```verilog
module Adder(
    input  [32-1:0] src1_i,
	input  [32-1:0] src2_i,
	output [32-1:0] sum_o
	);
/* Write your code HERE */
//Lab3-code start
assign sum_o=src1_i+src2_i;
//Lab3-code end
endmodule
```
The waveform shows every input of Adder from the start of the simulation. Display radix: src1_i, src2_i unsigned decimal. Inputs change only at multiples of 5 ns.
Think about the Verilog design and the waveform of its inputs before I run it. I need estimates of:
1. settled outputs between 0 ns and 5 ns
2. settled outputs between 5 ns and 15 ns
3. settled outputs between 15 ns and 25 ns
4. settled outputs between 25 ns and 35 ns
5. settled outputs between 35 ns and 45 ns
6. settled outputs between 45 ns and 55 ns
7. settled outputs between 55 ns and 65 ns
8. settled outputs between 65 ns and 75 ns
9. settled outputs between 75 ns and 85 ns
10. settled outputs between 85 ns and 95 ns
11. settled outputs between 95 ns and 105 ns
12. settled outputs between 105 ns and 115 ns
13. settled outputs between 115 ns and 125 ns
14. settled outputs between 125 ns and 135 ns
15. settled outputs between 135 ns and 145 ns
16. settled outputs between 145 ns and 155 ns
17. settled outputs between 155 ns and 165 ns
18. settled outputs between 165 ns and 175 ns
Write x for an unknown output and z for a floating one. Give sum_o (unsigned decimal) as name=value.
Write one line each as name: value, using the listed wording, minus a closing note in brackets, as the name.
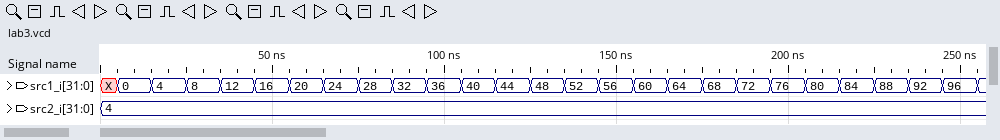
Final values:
settled outputs between 0 ns and 5 ns: sum_o=x
settled outputs between 5 ns and 15 ns: sum_o=4
settled outputs between 15 ns and 25 ns: sum_o=8
settled outputs between 25 ns and 35 ns: sum_o=12
settled outputs between 35 ns and 45 ns: sum_o=16
settled outputs between 45 ns and 55 ns: sum_o=20
settled outputs between 55 ns and 65 ns: sum_o=24
settled outputs between 65 ns and 75 ns: sum_o=28
settled outputs between 75 ns and 85 ns: sum_o=32
settled outputs between 85 ns and 95 ns: sum_o=36
settled outputs between 95 ns and 105 ns: sum_o=40
settled outputs between 105 ns and 115 ns: sum_o=44
settled outputs between 115 ns and 125 ns: sum_o=48
settled outputs between 125 ns and 135 ns: sum_o=52
settled outputs between 135 ns and 145 ns: sum_o=56
settled outputs between 145 ns and 155 ns: sum_o=60
settled outputs between 155 ns and 165 ns: sum_o=64
settled outputs between 165 ns and 175 ns: sum_o=68
